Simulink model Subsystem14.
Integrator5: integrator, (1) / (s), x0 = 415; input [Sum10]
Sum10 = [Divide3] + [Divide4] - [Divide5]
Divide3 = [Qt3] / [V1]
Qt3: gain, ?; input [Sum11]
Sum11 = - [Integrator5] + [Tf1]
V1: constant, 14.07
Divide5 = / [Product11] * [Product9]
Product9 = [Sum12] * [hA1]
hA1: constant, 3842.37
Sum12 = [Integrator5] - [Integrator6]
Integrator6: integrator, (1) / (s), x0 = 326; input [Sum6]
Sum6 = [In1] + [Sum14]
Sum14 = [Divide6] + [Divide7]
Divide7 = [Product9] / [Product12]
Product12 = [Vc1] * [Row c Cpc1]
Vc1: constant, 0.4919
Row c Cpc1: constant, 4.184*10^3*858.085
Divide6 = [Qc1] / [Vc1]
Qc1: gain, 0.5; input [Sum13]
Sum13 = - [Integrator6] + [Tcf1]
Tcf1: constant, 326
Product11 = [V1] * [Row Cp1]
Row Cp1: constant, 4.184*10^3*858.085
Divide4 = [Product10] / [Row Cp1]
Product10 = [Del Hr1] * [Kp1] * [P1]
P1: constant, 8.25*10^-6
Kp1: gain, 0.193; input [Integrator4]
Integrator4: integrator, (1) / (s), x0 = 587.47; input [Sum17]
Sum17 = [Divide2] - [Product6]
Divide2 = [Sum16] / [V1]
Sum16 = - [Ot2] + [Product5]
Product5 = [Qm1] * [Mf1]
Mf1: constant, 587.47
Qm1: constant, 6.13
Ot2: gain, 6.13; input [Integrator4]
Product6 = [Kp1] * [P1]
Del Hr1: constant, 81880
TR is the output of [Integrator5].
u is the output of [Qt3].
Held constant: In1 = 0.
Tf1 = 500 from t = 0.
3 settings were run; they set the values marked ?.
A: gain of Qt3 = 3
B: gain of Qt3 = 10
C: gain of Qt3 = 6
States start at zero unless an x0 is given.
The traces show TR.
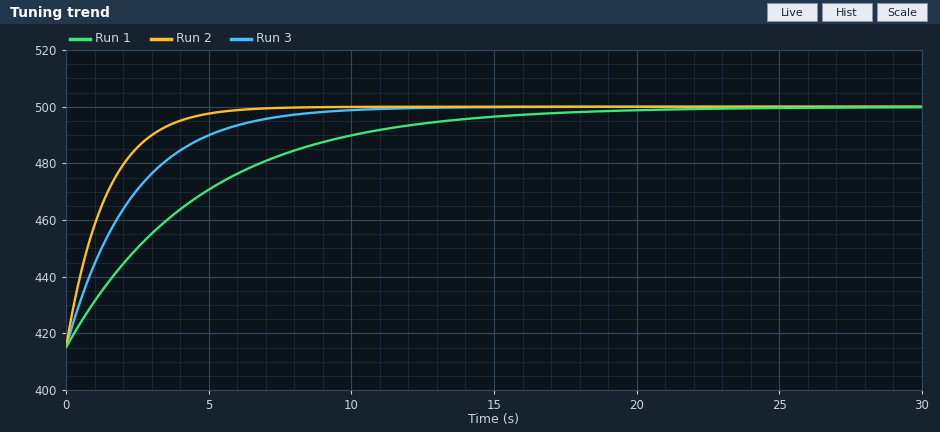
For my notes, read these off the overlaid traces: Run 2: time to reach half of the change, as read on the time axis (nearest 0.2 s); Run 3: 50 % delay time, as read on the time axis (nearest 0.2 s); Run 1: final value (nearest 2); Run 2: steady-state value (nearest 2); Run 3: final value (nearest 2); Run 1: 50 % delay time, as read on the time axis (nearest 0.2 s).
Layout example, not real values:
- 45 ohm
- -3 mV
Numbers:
- 1.0 s
- 1.6 s
- 500
- 500
- 500
- 3.2 s
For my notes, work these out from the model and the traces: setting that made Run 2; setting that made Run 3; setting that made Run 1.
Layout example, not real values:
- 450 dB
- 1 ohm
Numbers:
- B
- C
- A
